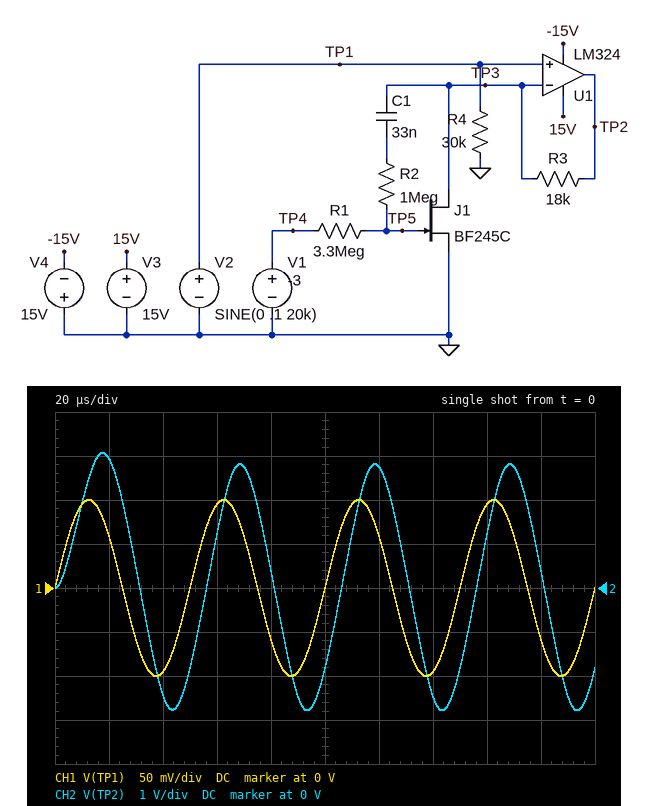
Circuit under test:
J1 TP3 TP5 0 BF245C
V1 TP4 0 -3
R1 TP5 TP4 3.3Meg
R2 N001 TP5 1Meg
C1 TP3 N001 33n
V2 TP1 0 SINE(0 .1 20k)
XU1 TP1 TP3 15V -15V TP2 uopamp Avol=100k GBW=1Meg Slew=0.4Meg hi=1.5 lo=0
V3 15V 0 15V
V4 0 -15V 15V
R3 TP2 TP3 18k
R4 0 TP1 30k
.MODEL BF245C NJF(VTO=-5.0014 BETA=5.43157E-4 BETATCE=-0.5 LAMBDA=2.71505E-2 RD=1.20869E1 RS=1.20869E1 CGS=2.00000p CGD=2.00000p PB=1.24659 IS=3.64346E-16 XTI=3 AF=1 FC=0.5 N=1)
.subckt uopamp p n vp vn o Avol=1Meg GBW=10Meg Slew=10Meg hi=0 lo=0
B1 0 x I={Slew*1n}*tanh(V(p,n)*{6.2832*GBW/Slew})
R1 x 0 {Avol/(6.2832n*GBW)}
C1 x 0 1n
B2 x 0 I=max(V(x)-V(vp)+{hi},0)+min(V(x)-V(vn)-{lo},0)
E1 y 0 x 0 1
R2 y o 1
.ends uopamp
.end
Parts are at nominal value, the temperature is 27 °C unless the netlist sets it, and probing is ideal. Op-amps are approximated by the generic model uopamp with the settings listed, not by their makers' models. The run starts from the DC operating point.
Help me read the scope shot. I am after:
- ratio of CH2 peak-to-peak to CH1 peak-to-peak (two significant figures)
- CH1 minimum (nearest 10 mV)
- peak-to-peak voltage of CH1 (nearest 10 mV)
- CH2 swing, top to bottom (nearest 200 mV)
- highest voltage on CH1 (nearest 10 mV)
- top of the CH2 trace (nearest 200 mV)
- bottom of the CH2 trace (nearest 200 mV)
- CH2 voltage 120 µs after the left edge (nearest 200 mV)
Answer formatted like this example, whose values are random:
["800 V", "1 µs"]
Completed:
["29", "-100 mV", "200 mV", "5.8 V", "100 mV", "3.0 V", "-2.8 V", "2.8 V"]
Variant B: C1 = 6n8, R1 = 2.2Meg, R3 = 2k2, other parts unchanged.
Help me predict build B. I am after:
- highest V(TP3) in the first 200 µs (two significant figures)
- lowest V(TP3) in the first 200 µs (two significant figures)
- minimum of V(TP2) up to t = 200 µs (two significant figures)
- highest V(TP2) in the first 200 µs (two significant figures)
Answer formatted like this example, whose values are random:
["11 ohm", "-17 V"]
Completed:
["99 mV", "-99 mV", "-550 mV", "560 mV"]
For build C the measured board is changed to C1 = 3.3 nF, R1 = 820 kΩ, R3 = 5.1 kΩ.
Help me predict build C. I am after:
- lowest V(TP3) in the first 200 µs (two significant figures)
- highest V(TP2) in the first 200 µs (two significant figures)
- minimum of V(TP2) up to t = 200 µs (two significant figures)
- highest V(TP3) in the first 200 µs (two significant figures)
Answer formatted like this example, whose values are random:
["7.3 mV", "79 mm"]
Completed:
["-97 mV", "1.1 V", "-1.1 V", "97 mV"]
